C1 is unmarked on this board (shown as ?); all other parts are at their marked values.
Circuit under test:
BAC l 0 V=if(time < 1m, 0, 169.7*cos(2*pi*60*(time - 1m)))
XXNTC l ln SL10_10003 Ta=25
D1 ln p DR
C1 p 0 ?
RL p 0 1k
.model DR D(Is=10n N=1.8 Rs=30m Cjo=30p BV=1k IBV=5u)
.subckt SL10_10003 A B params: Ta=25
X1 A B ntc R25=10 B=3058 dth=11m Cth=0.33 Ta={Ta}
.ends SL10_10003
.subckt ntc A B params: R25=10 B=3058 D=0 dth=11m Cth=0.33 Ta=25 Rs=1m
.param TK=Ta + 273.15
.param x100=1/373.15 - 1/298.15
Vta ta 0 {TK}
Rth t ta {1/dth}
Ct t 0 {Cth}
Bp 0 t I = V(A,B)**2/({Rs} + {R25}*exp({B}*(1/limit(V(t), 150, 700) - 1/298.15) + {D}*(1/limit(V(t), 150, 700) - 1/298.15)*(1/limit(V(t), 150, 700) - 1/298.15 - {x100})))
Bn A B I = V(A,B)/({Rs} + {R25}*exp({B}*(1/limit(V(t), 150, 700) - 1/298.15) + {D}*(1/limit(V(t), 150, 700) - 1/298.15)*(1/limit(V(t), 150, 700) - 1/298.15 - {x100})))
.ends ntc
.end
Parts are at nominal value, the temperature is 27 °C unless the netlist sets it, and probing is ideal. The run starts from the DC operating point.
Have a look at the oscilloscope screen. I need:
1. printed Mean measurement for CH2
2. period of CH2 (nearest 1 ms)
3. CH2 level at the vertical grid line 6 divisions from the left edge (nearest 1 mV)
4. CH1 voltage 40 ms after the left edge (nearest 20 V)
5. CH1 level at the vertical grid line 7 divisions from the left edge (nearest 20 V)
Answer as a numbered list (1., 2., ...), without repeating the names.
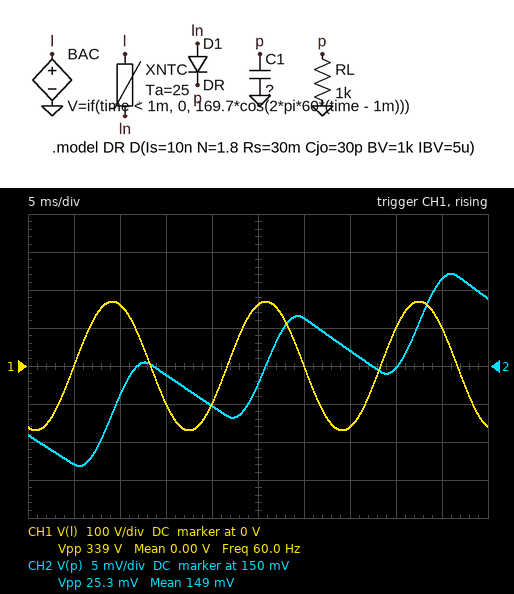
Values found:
1. 149 mV
2. 14 ms
3. 156 mV
4. 100 V
5. -160 V
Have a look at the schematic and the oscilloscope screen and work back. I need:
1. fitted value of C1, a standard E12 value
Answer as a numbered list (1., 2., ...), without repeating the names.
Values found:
1. 180 µF
